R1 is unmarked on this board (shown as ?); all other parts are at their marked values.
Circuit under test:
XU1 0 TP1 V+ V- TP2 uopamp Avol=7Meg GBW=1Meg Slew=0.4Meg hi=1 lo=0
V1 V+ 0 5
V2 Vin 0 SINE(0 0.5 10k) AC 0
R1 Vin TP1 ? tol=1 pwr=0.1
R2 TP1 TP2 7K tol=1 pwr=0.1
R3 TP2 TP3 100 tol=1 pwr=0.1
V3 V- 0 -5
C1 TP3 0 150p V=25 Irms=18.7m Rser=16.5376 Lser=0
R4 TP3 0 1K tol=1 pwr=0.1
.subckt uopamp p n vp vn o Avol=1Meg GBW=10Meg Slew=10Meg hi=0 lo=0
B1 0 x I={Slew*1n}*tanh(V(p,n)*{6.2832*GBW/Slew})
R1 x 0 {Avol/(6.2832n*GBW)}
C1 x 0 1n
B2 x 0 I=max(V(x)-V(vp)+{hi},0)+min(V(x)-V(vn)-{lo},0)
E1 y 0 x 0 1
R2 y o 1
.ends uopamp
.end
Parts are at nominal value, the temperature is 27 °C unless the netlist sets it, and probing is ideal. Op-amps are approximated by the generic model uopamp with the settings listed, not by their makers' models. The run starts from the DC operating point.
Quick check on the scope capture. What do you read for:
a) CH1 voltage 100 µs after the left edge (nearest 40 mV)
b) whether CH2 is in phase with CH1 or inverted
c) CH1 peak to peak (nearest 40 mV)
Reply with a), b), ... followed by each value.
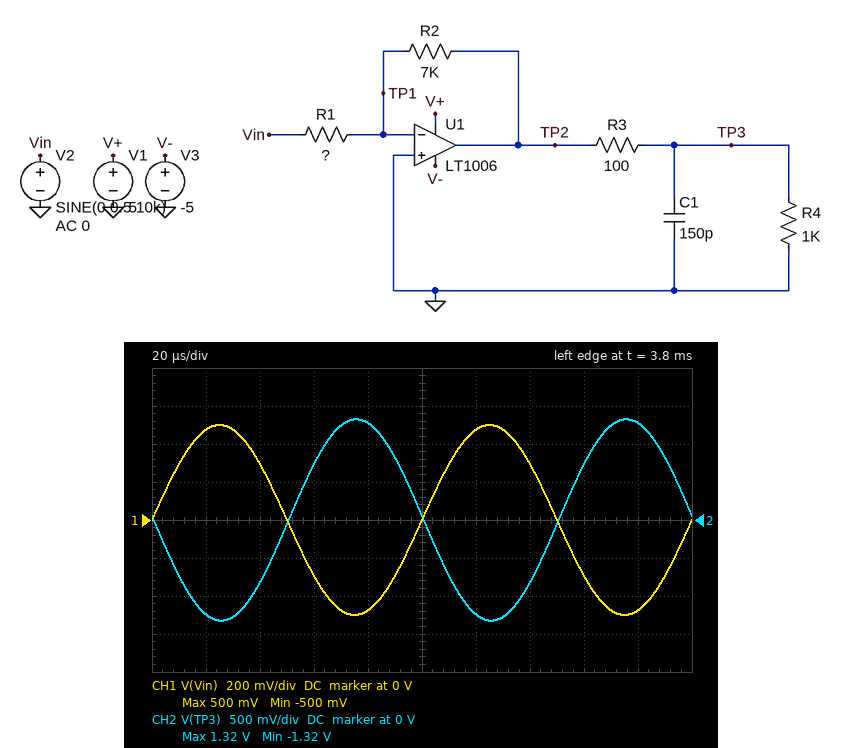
a) 0 V
b) inverted
c) 1.00 V
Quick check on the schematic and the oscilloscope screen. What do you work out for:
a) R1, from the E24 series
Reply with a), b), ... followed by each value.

a) 2.4 kΩ
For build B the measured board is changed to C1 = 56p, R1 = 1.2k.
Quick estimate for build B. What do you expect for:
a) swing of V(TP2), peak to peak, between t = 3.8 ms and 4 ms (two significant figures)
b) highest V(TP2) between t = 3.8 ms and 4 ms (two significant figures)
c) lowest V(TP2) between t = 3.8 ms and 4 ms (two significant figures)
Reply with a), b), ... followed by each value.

a) 5.8 V
b) 2.9 V
c) -2.9 V
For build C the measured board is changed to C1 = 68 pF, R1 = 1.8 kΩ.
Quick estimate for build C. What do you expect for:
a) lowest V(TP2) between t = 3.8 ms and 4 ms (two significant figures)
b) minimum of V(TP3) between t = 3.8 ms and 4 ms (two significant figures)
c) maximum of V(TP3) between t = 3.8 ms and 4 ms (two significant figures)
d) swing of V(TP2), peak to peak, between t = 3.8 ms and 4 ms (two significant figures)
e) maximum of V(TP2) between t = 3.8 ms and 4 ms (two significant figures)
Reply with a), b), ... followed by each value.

a) -1.9 V
b) -1.8 V
c) 1.8 V
d) 3.9 V
e) 1.9 V
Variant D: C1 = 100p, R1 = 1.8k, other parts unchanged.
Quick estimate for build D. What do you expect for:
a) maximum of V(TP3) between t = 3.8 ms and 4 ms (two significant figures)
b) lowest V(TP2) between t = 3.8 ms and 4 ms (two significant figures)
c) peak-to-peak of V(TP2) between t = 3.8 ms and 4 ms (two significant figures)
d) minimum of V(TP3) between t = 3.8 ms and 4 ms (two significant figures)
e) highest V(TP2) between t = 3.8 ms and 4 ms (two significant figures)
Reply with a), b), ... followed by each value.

a) 1.8 V
b) -1.9 V
c) 3.9 V
d) -1.8 V
e) 1.9 V
